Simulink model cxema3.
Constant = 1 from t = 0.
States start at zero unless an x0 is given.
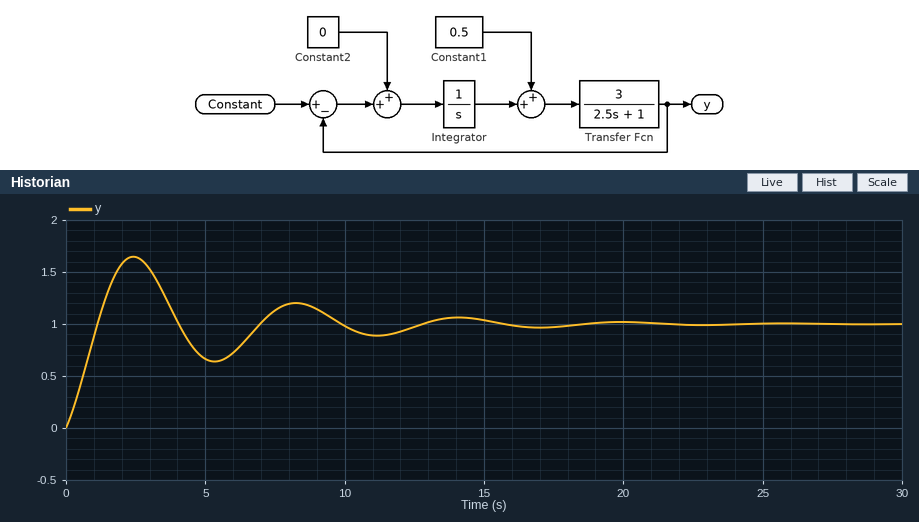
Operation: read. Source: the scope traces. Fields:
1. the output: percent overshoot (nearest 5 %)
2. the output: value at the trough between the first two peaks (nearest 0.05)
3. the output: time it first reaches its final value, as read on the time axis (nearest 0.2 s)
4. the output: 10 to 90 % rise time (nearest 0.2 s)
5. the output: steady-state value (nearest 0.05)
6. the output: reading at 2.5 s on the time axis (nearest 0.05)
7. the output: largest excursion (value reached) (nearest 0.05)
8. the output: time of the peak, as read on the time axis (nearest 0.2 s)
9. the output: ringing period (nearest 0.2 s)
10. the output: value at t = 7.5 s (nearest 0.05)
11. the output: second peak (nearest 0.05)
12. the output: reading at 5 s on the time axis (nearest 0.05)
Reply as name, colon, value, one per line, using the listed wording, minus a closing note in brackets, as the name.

the output: percent overshoot: 65 %
the output: value at the trough between the first two peaks: 0.65
the output: time it first reaches its final value, as read on the time axis: 1.2 s
the output: 10 to 90 % rise time: 0.8 s
the output: steady-state value: 1.00
the output: reading at 2.5 s on the time axis: 1.65
the output: largest excursion (value reached): 1.65
the output: time of the peak, as read on the time axis: 2.4 s
the output: ringing period: 5.8 s
the output: value at t = 7.5 s: 1.15
the output: second peak: 1.20
the output: reading at 5 s on the time axis: 0.65
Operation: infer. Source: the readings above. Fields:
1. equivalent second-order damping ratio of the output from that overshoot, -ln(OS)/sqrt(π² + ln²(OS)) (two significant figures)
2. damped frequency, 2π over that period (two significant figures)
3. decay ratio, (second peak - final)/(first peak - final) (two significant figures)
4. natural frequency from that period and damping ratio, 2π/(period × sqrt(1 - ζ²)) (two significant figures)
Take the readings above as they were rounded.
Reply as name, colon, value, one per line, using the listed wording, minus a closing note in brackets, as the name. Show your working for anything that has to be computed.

equivalent second-order damping ratio of the output from that overshoot, -ln(OS)/sqrt(π² + ln²(OS)): ln(0.65) = -0.431; 0.431 / sqrt(9.870 + 0.186) = 0.14
damped frequency, 2π over that period: 2π / 5.8 = 1.1 rad/s
decay ratio, (second peak - final)/(first peak - final): (1.2 - 1) / (1.65 - 1) = 0.31
natural frequency from that period and damping ratio, 2π/(period × sqrt(1 - ζ²)): 2π / (5.8 × sqrt(1 - 0.14²)) = 1.1 rad/s
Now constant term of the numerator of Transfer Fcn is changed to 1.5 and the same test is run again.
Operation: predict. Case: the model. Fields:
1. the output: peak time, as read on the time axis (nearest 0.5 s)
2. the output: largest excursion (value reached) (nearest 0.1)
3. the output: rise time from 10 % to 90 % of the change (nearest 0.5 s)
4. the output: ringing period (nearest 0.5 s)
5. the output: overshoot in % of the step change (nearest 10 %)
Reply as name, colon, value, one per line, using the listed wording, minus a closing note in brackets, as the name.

the output: peak time, as read on the time axis: 3.5 s
the output: largest excursion (value reached): 1.5
the output: rise time from 10 % to 90 % of the change: 1.5 s
the output: ringing period: 8.5 s
the output: overshoot in % of the step change: 50 %
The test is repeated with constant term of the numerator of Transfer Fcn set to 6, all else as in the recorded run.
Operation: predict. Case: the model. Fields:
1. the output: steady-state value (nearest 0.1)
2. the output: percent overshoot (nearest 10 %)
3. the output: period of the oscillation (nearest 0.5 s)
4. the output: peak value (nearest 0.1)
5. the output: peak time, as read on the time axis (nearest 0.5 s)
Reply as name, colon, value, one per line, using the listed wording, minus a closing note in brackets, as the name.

the output: steady-state value: 1.0
the output: percent overshoot: 90 %
the output: period of the oscillation: 4.0 s
the output: peak value: 1.9
the output: peak time, as read on the time axis: 1.5 s
